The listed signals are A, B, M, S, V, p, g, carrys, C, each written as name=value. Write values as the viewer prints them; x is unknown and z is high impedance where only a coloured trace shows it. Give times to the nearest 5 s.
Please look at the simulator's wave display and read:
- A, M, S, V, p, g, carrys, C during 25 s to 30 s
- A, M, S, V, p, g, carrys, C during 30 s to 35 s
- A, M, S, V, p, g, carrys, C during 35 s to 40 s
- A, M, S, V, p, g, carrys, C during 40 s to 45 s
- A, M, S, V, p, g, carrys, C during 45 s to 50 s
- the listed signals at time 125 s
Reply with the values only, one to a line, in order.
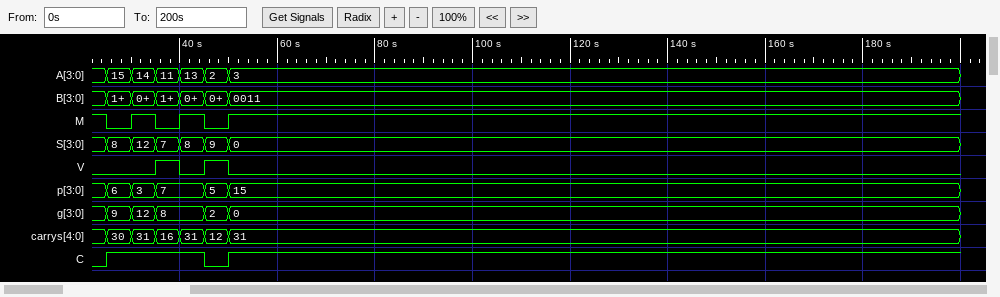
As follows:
A=15, M=0, S=8, V=0, p=6, g=9, carrys=30, C=1
A=14, M=1, S=12, V=0, p=3, g=12, carrys=31, C=1
A=11, M=0, S=7, V=1, p=7, g=8, carrys=16, C=1
A=13, M=1, S=8, V=0, p=7, g=8, carrys=31, C=1
A=2, M=0, S=9, V=1, p=5, g=2, carrys=12, C=0
A=3, B=0011, M=1, S=0, V=0, p=15, g=0, carrys=31, C=1
